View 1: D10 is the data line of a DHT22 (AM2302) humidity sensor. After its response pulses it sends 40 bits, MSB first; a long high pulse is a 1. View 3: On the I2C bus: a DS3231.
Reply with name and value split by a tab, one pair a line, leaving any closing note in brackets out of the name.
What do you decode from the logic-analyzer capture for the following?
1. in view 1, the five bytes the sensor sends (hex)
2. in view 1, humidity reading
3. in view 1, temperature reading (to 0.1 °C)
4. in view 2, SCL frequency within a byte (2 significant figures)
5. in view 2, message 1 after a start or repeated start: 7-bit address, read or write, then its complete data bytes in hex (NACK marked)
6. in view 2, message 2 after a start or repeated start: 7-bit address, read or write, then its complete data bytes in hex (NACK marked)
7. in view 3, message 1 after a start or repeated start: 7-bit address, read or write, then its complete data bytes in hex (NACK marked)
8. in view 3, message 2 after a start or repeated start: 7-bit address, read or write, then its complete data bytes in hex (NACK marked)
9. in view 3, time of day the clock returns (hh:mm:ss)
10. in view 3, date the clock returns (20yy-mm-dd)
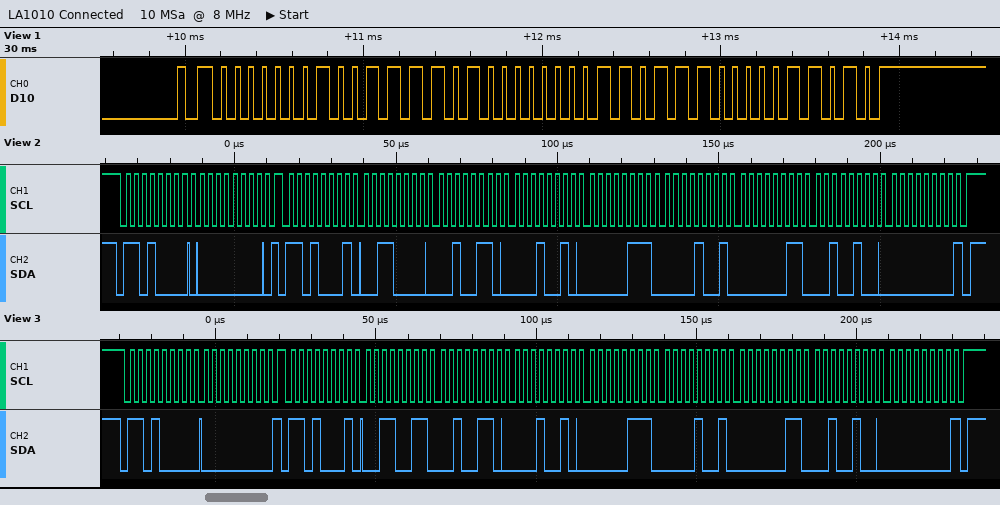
in view 1, the five bytes the sensor sends	01 3D 00 DC 1A
in view 1, humidity reading	31.7 %
in view 1, temperature reading	22.0 °C
in view 2, SCL frequency within a byte	400 kHz
in view 2, message 1 after a start or repeated start: 7-bit address, read or write, then its complete data bytes in hex	0x68 write: 00
in view 2, message 2 after a start or repeated start: 7-bit address, read or write, then its complete data bytes in hex	0x68 read: 30 26 12 07 09 03 24 00 NACK
in view 3, message 1 after a start or repeated start: 7-bit address, read or write, then its complete data bytes in hex	0x68 write: 00
in view 3, message 2 after a start or repeated start: 7-bit address, read or write, then its complete data bytes in hex	0x68 read: 33 26 12 07 09 03 24 00 NACK
in view 3, time of day the clock returns	12:26:33
in view 3, date the clock returns	2024-03-09
